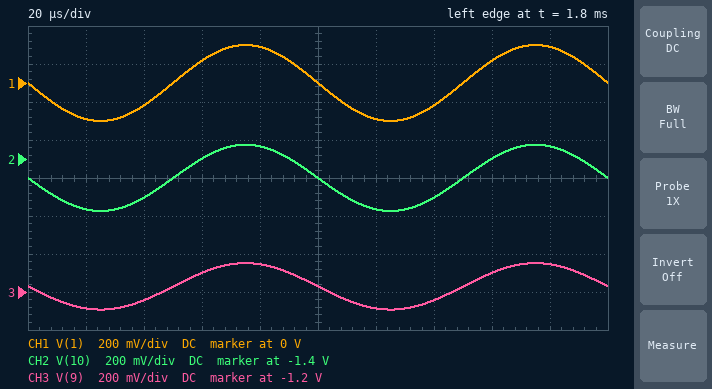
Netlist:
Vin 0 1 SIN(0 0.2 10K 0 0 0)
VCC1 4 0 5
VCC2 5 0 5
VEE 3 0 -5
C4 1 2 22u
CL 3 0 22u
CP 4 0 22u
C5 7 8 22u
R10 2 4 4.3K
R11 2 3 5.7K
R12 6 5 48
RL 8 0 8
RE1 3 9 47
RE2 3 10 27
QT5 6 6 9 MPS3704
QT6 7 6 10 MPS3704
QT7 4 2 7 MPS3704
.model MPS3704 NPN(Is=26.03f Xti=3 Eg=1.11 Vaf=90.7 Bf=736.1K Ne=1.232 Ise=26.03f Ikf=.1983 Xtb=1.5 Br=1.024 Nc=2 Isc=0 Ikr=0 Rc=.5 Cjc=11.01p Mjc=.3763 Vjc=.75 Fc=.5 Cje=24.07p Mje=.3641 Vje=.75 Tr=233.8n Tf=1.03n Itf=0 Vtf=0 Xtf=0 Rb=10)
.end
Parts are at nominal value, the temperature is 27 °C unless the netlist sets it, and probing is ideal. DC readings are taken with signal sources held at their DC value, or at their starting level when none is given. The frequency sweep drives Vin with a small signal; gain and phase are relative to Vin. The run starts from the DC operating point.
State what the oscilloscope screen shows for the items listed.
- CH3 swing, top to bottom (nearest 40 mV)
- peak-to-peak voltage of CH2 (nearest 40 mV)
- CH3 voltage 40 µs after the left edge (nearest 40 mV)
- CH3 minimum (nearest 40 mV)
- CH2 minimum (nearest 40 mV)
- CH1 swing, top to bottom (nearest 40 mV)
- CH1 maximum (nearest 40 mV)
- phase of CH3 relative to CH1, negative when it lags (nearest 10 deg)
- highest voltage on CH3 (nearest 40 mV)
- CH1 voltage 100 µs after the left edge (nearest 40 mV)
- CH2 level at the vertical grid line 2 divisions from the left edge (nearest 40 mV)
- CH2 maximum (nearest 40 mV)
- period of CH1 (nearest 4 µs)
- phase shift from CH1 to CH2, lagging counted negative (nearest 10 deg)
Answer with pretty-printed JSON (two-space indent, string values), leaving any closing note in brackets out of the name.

{
  "CH3 swing, top to bottom": "240 mV",
  "peak-to-peak voltage of CH2": "360 mV",
  "CH3 voltage 40 µs after the left edge": "-1.24 V",
  "CH3 minimum": "-1.28 V",
  "CH2 minimum": "-1.68 V",
  "CH1 swing, top to bottom": "400 mV",
  "CH1 maximum": "200 mV",
  "phase of CH3 relative to CH1, negative when it lags": "0 deg",
  "highest voltage on CH3": "-1.04 V",
  "CH1 voltage 100 µs after the left edge": "0 V",
  "CH2 level at the vertical grid line 2 divisions from the left edge": "-1.60 V",
  "CH2 maximum": "-1.32 V",
  "period of CH1": "100 µs",
  "phase shift from CH1 to CH2, lagging counted negative": "0 deg"
}
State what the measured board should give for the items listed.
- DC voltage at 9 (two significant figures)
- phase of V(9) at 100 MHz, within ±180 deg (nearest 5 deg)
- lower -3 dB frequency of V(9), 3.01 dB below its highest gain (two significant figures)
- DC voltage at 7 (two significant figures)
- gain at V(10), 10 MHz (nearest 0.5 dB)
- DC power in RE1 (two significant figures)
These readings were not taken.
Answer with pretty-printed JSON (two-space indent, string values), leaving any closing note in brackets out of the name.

{
  "DC voltage at 9": "-1.2 V",
  "phase of V(9) at 100 MHz, within ±180 deg": "150 deg",
  "lower -3 dB frequency of V(9), 3.01 dB below its highest gain": "5.6 Hz",
  "DC voltage at 7": "-1.4 V",
  "gain at V(10), 10 MHz": "-1.0 dB",
  "DC power in RE1": "310 mW"
}
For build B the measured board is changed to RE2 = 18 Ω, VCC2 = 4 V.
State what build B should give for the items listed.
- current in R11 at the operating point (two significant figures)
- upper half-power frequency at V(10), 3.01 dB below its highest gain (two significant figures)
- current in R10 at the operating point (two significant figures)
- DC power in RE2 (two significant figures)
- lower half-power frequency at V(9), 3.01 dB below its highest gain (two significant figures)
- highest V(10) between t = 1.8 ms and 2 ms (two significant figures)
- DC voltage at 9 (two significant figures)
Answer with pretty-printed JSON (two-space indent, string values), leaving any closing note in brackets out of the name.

{
  "current in R11 at the operating point": "680 µA",
  "upper half-power frequency at V(10), 3.01 dB below its highest gain": "59 MHz",
  "current in R10 at the operating point": "1.4 mA",
  "DC power in RE2": "490 mW",
  "lower half-power frequency at V(9), 3.01 dB below its highest gain": "6.5 Hz",
  "highest V(10) between t = 1.8 ms and 2 ms": "-1.9 V",
  "DC voltage at 9": "-1.7 V"
}
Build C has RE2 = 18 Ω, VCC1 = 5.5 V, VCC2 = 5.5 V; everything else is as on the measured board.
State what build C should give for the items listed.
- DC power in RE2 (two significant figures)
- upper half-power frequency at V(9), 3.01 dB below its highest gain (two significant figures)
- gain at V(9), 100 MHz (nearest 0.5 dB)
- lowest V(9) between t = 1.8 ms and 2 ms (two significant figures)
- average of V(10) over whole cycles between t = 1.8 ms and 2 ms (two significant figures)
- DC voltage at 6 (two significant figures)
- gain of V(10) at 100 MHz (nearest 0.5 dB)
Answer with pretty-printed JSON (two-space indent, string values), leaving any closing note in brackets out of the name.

{
  "DC power in RE2": "580 mW",
  "upper half-power frequency at V(9), 3.01 dB below its highest gain": "55 MHz",
  "gain at V(9), 100 MHz": "-9.5 dB",
  "lowest V(9) between t = 1.8 ms and 2 ms": "-1.4 V",
  "average of V(10) over whole cycles between t = 1.8 ms and 2 ms": "-1.8 V",
  "DC voltage at 6": "-520 mV",
  "gain of V(10) at 100 MHz": "-6.0 dB"
}
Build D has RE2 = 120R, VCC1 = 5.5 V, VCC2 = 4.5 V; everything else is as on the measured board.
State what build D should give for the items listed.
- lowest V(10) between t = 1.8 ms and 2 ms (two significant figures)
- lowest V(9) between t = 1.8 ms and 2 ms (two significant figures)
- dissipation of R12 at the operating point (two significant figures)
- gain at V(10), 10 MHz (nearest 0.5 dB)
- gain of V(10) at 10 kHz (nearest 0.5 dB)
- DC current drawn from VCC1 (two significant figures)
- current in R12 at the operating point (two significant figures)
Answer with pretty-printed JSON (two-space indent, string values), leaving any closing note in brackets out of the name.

{
  "lowest V(10) between t = 1.8 ms and 2 ms": "-650 mV",
  "lowest V(9) between t = 1.8 ms and 2 ms": "-680 mV",
  "dissipation of R12 at the operating point": "410 mW",
  "gain at V(10), 10 MHz": "-31.5 dB",
  "gain of V(10) at 10 kHz": "-68.5 dB",
  "DC current drawn from VCC1": "37 mA",
  "current in R12 at the operating point": "92 mA"
}
